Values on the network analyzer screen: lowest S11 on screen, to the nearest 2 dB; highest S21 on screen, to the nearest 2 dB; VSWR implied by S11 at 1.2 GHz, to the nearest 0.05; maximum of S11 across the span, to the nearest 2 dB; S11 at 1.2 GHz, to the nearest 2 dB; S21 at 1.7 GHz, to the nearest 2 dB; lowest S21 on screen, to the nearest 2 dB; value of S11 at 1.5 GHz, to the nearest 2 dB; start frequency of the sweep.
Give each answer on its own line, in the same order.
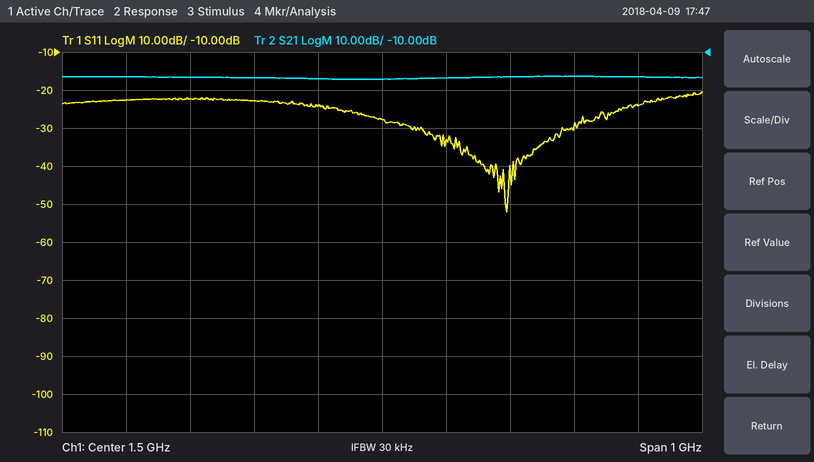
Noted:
-52 dB
-16 dB
1.15
-20 dB
-22 dB
-16 dB
-18 dB
-28 dB
1 GHz
